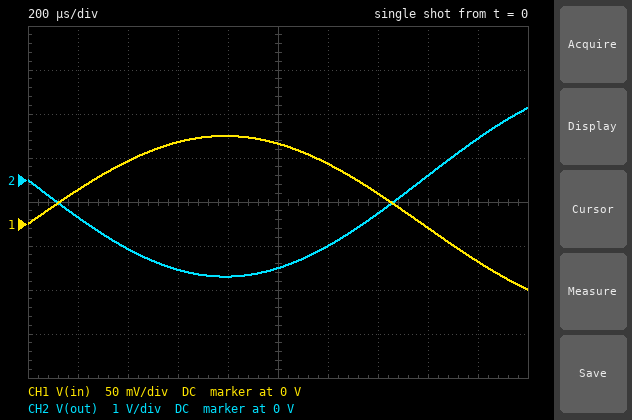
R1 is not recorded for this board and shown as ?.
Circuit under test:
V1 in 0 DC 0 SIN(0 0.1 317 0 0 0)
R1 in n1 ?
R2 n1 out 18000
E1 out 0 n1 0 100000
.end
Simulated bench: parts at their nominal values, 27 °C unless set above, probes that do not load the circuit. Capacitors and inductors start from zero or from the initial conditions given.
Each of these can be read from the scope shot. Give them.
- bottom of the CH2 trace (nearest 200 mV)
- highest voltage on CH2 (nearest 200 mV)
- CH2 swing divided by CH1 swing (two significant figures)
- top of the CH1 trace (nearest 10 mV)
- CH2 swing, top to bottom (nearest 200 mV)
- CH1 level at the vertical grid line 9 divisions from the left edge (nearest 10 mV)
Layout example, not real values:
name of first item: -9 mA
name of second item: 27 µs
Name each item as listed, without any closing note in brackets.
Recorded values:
bottom of the CH2 trace: -2.2 V
highest voltage on CH2: 1.6 V
CH2 swing divided by CH1 swing: 22
top of the CH1 trace: 100 mV
CH2 swing, top to bottom: 3.8 V
CH1 level at the vertical grid line 9 divisions from the left edge: -40 mV
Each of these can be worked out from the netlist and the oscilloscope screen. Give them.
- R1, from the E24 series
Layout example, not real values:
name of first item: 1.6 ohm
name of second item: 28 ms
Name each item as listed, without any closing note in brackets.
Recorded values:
R1, from the E24 series: 820 Ω
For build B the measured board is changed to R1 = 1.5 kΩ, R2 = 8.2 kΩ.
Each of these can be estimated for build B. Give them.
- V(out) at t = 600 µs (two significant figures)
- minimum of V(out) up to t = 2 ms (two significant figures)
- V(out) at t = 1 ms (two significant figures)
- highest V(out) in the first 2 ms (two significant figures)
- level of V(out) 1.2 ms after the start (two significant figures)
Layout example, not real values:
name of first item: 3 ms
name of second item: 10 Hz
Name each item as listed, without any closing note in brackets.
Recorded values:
V(out) at t = 600 µs: -510 mV
minimum of V(out) up to t = 2 ms: -550 mV
V(out) at t = 1 ms: -500 mV
highest V(out) in the first 2 ms: 410 mV
level of V(out) 1.2 ms after the start: -370 mV
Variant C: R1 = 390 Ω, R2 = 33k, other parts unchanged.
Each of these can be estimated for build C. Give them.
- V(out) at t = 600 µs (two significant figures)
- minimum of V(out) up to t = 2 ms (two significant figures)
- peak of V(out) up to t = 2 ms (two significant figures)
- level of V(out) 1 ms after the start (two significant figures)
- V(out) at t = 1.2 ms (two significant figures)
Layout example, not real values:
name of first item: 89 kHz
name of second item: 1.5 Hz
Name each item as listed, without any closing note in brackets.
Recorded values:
V(out) at t = 600 µs: -7.9 V
minimum of V(out) up to t = 2 ms: -8.5 V
peak of V(out) up to t = 2 ms: 6.3 V
level of V(out) 1 ms after the start: -7.7 V
V(out) at t = 1.2 ms: -5.8 V
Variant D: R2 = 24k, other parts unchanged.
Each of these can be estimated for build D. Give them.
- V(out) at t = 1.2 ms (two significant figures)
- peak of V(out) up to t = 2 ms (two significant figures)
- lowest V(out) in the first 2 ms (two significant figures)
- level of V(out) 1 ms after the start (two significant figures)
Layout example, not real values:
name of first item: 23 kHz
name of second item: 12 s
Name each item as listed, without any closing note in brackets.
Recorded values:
V(out) at t = 1.2 ms: -2.0 V
peak of V(out) up to t = 2 ms: 2.2 V
lowest V(out) in the first 2 ms: -2.9 V
level of V(out) 1 ms after the start: -2.7 V
